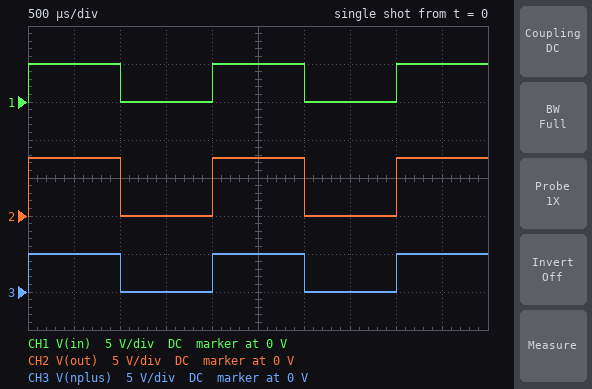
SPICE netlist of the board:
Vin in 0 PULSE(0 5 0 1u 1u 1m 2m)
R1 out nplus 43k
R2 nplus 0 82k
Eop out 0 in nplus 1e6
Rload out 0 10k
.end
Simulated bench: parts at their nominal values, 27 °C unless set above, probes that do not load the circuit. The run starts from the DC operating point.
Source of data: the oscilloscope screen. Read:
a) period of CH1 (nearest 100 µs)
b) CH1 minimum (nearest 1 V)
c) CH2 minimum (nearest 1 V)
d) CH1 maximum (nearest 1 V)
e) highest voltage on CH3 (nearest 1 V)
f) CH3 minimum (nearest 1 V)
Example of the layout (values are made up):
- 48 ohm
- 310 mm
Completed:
- 2.0 ms
- 0 V
- 0 V
- 5 V
- 5 V
- 0 V
